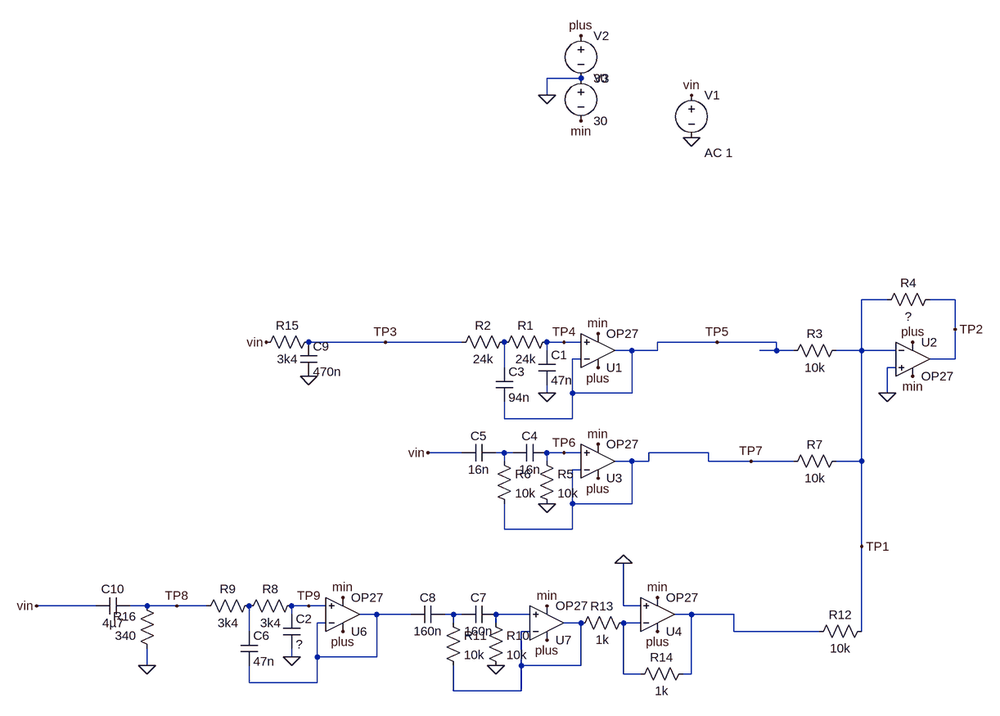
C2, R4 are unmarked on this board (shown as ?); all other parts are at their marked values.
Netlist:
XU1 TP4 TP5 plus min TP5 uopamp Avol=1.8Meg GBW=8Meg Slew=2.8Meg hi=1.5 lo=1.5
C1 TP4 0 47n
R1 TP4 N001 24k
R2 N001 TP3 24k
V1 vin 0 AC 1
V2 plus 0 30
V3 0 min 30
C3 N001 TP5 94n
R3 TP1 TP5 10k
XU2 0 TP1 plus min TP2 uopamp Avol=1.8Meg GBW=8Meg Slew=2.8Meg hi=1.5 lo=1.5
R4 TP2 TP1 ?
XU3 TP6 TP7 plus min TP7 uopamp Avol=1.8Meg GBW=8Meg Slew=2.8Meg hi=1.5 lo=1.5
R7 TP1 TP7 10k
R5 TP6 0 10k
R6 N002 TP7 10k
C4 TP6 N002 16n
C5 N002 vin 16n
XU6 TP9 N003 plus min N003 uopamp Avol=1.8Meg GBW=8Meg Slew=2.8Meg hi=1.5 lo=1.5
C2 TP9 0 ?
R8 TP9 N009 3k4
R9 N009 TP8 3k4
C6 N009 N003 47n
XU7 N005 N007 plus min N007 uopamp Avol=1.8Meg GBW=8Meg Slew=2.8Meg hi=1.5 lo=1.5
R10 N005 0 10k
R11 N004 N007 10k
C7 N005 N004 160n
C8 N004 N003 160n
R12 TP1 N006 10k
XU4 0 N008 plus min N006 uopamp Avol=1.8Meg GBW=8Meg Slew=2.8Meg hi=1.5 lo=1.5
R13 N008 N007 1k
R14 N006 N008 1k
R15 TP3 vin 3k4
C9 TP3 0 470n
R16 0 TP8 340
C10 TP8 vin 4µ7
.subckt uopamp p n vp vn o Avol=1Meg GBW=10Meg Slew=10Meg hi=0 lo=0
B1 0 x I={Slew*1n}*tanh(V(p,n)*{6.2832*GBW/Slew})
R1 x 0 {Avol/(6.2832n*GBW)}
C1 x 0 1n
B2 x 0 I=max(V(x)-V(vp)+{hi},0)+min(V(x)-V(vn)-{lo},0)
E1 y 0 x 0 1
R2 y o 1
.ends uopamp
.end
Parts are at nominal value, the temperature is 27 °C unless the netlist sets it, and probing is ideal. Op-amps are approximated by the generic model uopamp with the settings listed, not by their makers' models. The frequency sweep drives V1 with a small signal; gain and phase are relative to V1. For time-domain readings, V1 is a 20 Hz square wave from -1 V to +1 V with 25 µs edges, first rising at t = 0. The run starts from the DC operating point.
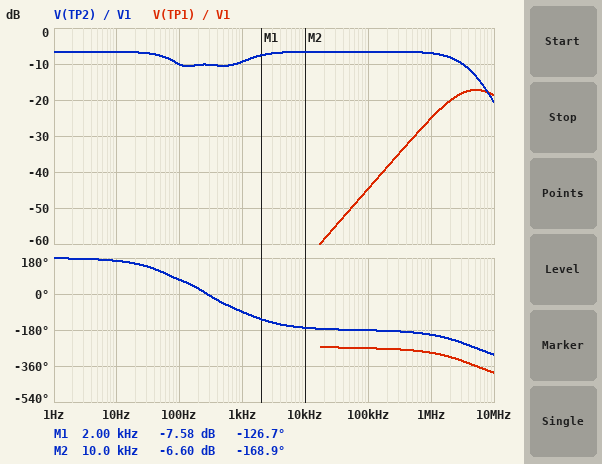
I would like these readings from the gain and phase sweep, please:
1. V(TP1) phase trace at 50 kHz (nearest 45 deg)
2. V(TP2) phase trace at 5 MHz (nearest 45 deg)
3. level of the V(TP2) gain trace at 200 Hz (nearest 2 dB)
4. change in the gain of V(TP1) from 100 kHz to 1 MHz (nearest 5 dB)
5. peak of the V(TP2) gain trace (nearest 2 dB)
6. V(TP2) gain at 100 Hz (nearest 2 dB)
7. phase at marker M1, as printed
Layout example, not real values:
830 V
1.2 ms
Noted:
-270 deg
-270 deg
-10 dB
20 dB
-6 dB
-10 dB
-126.7 deg
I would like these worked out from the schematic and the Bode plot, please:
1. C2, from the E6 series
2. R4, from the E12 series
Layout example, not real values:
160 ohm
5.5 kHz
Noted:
100 nF
4.7 kΩ
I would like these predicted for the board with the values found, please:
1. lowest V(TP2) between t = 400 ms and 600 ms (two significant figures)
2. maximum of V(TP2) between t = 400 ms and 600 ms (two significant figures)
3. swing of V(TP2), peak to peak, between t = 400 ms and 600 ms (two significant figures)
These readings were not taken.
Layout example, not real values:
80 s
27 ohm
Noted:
-850 mV
850 mV
1.7 V
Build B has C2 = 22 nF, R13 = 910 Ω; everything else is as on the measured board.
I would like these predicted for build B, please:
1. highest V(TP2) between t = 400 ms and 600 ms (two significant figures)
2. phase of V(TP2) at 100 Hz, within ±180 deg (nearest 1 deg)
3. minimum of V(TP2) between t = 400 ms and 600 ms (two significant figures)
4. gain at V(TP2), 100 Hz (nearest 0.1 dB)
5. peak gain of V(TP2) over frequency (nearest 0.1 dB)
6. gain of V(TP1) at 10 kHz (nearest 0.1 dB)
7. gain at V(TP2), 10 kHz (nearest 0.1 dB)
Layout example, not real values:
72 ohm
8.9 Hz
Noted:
1.3 V
81 deg
-1.3 V
-10.6 dB
-3.5 dB
-64.5 dB
-6.4 dB
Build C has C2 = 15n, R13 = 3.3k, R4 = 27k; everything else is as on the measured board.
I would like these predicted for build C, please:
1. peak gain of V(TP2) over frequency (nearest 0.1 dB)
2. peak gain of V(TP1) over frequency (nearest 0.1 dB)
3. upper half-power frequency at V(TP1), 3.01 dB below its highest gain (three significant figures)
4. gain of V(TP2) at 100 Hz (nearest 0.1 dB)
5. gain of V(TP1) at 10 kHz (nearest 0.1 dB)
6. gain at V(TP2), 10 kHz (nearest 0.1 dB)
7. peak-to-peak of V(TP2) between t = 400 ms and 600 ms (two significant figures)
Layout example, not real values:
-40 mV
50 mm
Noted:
8.7 dB
-11.5 dB
9.61 MHz
2.3 dB
-49.4 dB
8.6 dB
9.5 V
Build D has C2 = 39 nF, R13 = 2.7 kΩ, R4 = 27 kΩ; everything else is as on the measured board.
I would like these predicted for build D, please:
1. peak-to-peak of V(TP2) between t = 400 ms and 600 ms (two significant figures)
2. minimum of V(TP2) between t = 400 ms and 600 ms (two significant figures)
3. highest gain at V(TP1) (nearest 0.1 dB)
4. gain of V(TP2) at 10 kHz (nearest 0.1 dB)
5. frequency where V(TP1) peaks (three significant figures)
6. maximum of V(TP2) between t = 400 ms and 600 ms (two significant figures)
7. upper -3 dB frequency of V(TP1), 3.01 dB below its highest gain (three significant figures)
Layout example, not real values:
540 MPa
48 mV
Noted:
9.0 V
-4.5 V
-11.5 dB
8.6 dB
2.65 MHz
4.5 V
9.61 MHz
